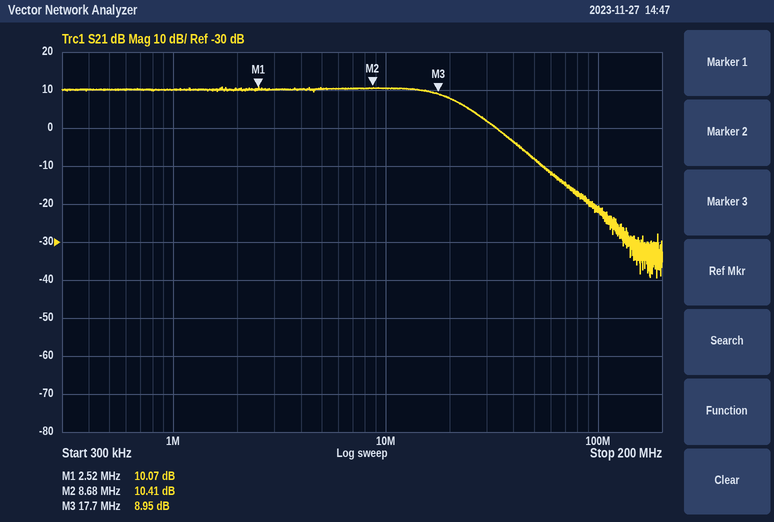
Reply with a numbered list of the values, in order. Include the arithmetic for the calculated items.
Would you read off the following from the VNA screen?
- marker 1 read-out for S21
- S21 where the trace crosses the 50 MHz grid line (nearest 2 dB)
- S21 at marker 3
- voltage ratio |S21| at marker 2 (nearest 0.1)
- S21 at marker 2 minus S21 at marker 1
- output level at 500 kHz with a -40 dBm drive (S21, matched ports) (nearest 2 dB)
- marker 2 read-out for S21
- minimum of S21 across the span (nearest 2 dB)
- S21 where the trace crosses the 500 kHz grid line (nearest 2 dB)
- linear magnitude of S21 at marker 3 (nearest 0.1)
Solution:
1. 10.07 dB
2. -8 dB
3. 8.95 dB
4. 10^(10.41/20) ≈ 3.3
5. 10.41 − (10.07) = 0.34 dB
6. -40 dBm + (10 dB) = -30 dBm
7. 10.41 dB
8. -40 dB
9. 10 dB
10. 10^(8.95/20) ≈ 2.8
